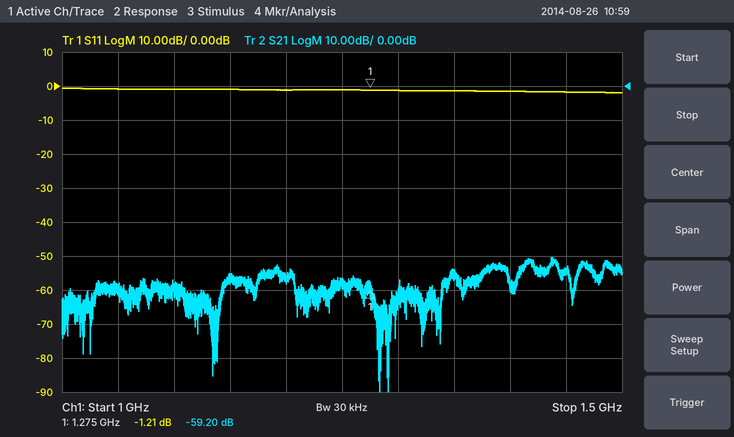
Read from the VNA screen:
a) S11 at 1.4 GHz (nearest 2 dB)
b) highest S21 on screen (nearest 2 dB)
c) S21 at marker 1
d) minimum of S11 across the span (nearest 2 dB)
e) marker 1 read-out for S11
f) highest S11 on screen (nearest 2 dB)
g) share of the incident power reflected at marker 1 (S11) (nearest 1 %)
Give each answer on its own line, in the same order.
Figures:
-2 dB
-50 dB
-59.20 dB
-2 dB
-1.21 dB
0 dB
76 %
